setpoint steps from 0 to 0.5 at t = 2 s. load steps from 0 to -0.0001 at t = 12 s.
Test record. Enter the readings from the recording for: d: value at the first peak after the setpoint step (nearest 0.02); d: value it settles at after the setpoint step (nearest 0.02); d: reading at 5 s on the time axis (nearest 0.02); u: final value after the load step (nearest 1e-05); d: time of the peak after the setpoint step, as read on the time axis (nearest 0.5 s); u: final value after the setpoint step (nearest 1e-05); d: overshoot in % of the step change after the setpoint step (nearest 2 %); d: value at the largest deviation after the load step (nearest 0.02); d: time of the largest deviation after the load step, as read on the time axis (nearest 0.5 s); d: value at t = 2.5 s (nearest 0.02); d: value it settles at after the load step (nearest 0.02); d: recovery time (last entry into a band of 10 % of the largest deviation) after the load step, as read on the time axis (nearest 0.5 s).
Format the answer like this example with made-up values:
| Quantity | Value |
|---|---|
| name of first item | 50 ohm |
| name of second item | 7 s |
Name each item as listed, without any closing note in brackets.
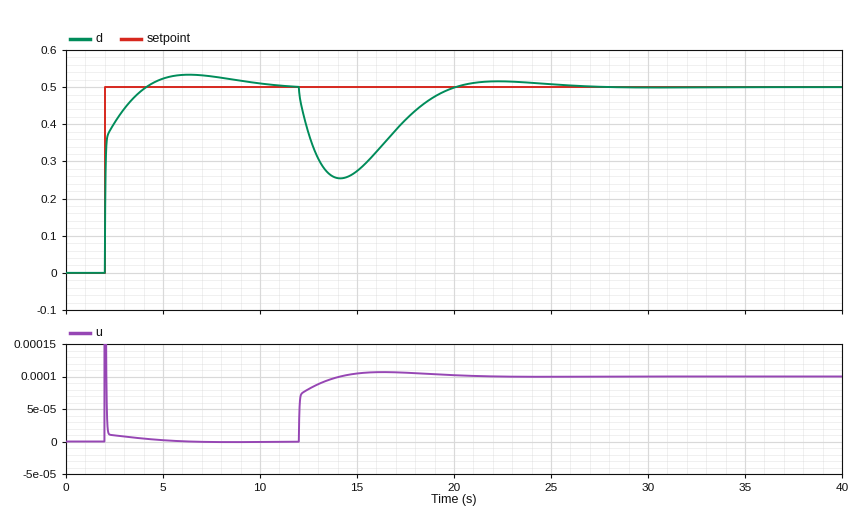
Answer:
| Quantity | Value |
|---|---|
| d: value at the first peak after the setpoint step | 0.54 |
| d: value it settles at after the setpoint step | 0.50 |
| d: reading at 5 s on the time axis | 0.52 |
| u: final value after the load step | 0.00010 |
| d: time of the peak after the setpoint step, as read on the time axis | 6.5 s |
| u: final value after the setpoint step | 0.00000 |
| d: overshoot in % of the step change after the setpoint step | 6 % |
| d: value at the largest deviation after the load step | 0.26 |
| d: time of the largest deviation after the load step, as read on the time axis | 14.0 s |
| d: value at t = 2.5 s | 0.40 |
| d: value it settles at after the load step | 0.50 |
| d: recovery time (last entry into a band of 10 % of the largest deviation) after the load step, as read on the time axis | 19.0 s |
